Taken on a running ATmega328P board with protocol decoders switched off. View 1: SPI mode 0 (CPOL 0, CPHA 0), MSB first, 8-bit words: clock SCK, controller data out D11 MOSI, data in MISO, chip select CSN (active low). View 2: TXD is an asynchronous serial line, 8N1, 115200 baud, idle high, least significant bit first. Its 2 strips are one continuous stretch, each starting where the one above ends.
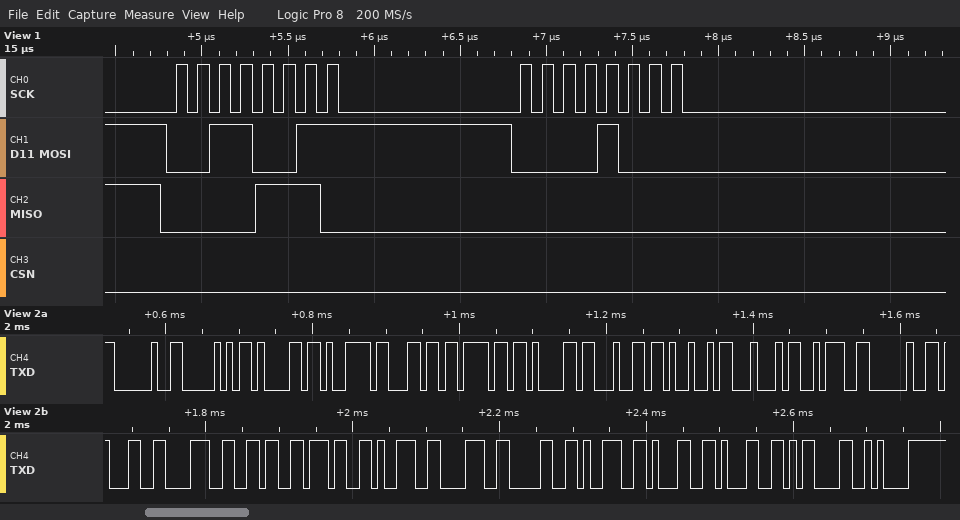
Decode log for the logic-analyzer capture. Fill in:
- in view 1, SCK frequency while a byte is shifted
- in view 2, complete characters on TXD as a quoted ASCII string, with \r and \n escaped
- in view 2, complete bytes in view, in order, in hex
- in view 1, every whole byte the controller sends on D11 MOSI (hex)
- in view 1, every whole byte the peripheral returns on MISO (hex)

8 MHz
" PayloadID: 1867980911\r\n"
20 50 61 79 6C 6F 61 64 49 44 3A 20 31 38 36 37 39 38 30 39 31 31 0D 0A
33 08
0E 00
